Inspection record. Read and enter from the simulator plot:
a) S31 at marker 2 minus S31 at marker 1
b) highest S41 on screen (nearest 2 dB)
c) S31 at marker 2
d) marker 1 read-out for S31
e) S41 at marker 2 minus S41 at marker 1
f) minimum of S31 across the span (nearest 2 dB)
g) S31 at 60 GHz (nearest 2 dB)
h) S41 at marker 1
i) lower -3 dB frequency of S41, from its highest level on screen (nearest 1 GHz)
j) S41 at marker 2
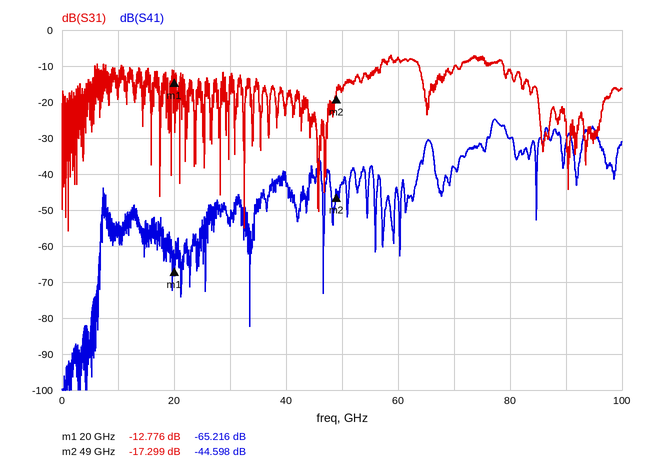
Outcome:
-4.523 dB
-24 dB
-17.299 dB
-12.776 dB
20.618 dB
-56 dB
-8 dB
-65.216 dB
77 GHz
-44.598 dB
